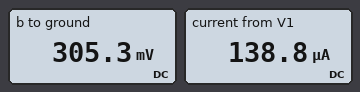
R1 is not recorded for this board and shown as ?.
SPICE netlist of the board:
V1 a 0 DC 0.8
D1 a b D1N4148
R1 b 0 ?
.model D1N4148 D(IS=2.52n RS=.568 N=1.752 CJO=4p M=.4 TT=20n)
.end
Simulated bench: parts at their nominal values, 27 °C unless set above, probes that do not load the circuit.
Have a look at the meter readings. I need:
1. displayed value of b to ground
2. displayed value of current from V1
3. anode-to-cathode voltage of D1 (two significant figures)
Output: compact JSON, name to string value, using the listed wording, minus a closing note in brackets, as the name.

{"displayed value of b to ground": "305.3 mV", "displayed value of current from V1": "138.8 µA", "anode-to-cathode voltage of D1": "490 mV"}
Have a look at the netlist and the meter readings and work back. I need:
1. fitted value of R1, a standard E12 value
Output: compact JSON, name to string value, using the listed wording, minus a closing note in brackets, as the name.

{"fitted value of R1, a standard E12 value": "2.2 kΩ"}
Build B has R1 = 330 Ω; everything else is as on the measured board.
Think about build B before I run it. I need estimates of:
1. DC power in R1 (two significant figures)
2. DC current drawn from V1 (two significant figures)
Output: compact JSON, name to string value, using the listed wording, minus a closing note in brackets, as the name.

{"DC power in R1": "160 µW", "DC current drawn from V1": "700 µA"}
